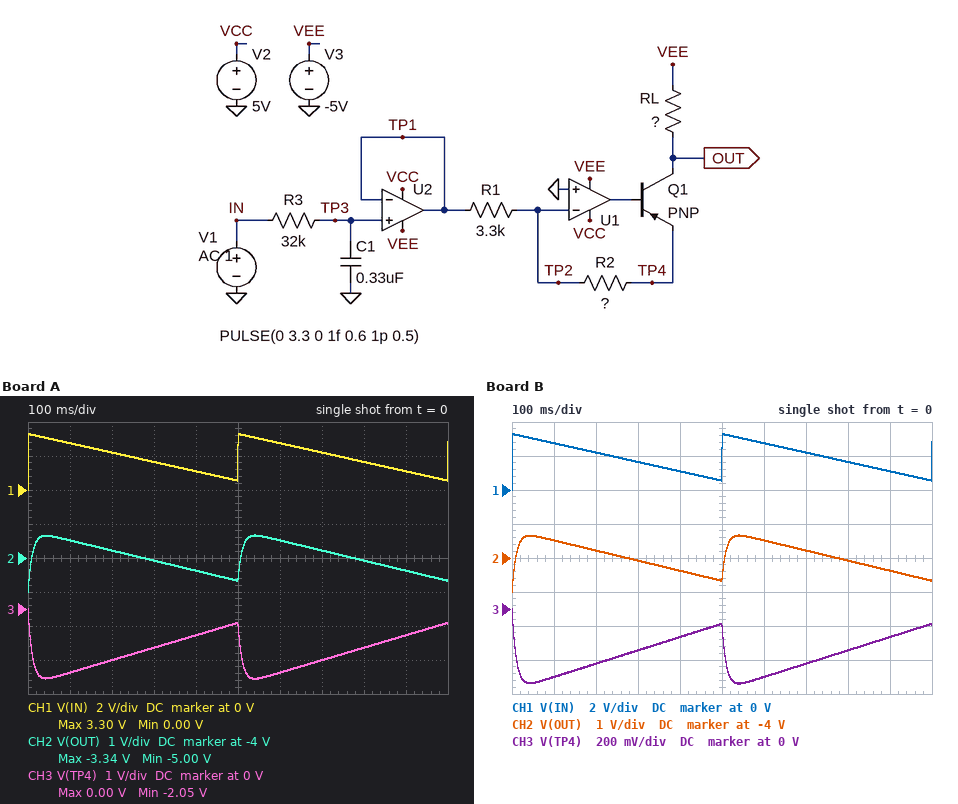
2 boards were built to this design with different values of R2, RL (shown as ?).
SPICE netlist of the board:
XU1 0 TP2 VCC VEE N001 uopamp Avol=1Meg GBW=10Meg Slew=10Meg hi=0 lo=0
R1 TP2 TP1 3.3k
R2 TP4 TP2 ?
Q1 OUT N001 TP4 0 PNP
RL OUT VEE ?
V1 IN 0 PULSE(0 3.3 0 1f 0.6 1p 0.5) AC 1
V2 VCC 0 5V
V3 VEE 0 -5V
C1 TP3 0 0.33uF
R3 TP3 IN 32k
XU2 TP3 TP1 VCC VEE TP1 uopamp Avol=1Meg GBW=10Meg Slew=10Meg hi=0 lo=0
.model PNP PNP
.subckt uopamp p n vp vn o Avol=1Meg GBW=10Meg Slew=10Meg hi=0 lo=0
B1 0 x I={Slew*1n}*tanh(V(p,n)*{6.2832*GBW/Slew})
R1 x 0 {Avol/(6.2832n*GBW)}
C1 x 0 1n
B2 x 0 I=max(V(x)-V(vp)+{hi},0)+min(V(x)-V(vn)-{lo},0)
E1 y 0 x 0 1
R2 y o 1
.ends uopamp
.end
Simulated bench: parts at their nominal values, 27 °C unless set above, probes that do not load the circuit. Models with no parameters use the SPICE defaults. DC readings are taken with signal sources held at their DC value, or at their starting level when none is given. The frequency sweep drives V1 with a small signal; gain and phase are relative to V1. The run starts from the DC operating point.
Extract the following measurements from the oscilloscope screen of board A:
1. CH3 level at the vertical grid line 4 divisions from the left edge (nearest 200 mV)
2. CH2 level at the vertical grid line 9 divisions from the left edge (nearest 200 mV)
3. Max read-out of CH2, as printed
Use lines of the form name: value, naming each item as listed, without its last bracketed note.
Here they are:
CH3 level at the vertical grid line 4 divisions from the left edge: -800 mV
CH2 level at the vertical grid line 9 divisions from the left edge: -4.4 V
Max read-out of CH2, as printed: -3.34 V
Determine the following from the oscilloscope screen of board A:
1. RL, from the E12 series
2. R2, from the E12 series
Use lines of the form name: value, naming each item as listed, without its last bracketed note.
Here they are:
RL, from the E12 series: 1.8 kΩ
R2, from the E12 series: 2.2 kΩ
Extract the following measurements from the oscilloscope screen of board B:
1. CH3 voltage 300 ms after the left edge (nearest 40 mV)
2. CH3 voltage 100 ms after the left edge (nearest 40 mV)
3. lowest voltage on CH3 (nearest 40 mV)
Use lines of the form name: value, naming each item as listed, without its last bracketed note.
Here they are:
CH3 voltage 300 ms after the left edge: -240 mV
CH3 voltage 100 ms after the left edge: -400 mV
lowest voltage on CH3: -440 mV
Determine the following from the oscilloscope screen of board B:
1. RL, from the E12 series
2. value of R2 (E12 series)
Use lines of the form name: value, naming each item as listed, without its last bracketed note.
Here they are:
RL, from the E12 series: 1.8 kΩ
value of R2: 470 Ω
